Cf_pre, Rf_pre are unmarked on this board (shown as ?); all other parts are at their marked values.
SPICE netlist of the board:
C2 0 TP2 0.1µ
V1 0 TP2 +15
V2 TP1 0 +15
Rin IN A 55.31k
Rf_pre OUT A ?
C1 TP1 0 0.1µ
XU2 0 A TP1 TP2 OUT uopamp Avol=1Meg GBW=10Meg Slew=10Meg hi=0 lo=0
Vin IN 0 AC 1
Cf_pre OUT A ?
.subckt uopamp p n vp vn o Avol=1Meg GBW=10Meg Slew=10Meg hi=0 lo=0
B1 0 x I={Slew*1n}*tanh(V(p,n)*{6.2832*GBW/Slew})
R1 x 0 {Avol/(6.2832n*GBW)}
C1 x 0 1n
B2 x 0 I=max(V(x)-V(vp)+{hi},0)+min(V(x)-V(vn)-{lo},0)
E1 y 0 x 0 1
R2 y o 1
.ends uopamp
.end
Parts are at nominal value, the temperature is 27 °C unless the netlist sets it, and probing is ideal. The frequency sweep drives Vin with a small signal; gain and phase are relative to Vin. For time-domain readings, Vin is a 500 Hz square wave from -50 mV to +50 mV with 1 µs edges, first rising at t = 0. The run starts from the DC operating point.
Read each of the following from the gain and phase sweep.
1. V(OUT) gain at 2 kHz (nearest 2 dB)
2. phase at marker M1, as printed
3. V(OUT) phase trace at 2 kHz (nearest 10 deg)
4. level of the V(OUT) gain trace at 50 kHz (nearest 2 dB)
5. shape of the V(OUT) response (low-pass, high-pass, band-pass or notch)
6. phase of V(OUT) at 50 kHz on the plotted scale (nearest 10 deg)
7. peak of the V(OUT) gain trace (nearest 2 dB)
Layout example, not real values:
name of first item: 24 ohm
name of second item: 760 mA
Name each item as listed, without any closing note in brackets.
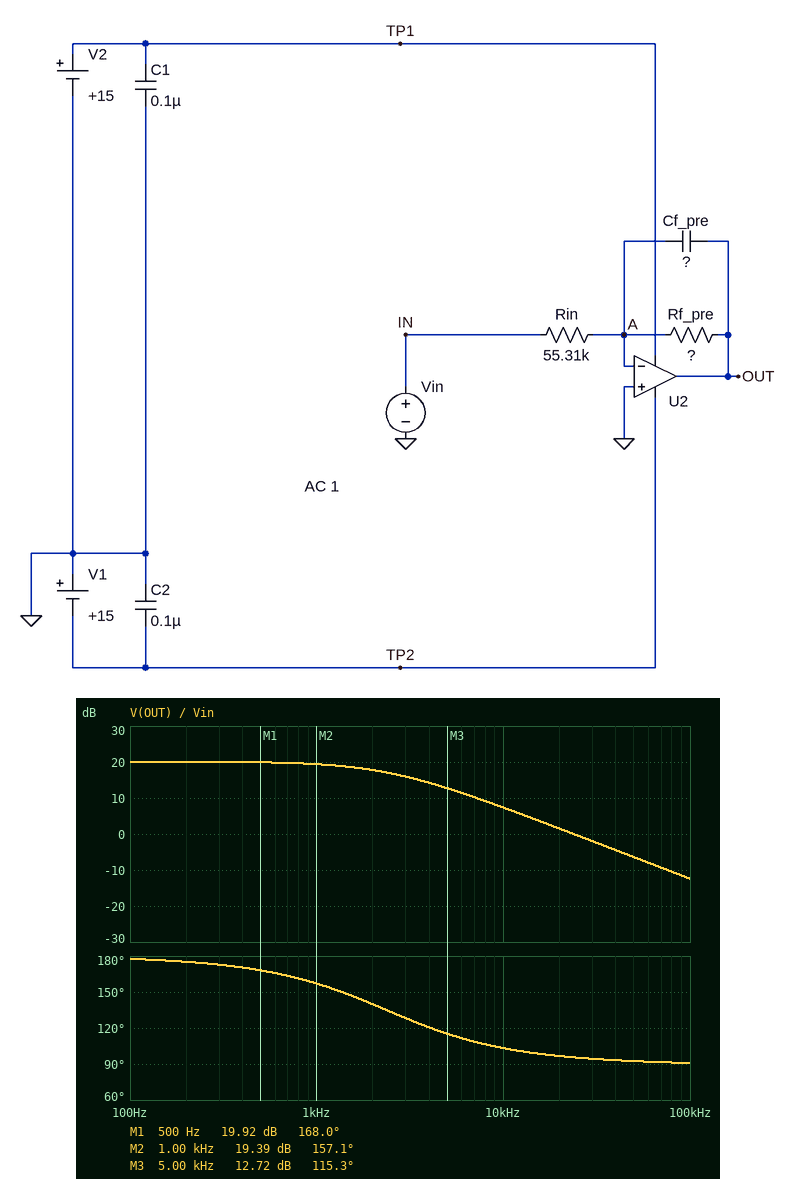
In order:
V(OUT) gain at 2 kHz: 18 dB
phase at marker M1, as printed: 168.0 deg
V(OUT) phase trace at 2 kHz: 140 deg
level of the V(OUT) gain trace at 50 kHz: -6 dB
shape of the V(OUT) response: low-pass
phase of V(OUT) at 50 kHz on the plotted scale: 90 deg
peak of the V(OUT) gain trace: 20 dB
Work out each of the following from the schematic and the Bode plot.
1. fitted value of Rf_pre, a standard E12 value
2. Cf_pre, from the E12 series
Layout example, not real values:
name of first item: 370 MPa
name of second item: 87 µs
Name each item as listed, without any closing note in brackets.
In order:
fitted value of Rf_pre, a standard E12 value: 560 kΩ
Cf_pre, from the E12 series: 120 pF
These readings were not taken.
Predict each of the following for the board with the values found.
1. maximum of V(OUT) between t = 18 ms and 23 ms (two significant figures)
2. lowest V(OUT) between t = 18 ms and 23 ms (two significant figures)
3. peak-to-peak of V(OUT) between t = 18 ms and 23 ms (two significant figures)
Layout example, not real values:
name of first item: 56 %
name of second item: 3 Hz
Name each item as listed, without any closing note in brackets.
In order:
maximum of V(OUT) between t = 18 ms and 23 ms: 510 mV
lowest V(OUT) between t = 18 ms and 23 ms: -510 mV
peak-to-peak of V(OUT) between t = 18 ms and 23 ms: 1.0 V
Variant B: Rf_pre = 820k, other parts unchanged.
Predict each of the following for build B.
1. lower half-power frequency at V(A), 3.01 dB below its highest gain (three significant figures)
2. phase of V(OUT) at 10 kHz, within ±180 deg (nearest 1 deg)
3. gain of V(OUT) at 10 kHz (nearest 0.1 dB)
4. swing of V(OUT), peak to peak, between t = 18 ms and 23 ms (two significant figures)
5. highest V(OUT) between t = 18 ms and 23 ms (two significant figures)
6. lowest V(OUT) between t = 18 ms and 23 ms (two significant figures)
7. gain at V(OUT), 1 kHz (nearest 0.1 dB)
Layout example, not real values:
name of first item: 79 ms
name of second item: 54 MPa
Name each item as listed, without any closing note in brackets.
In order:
lower half-power frequency at V(A), 3.01 dB below its highest gain: 1.61 kHz
phase of V(OUT) at 10 kHz, within ±180 deg: 99 deg
gain of V(OUT) at 10 kHz: 7.5 dB
swing of V(OUT), peak to peak, between t = 18 ms and 23 ms: 1.5 V
highest V(OUT) between t = 18 ms and 23 ms: 740 mV
lowest V(OUT) between t = 18 ms and 23 ms: -740 mV
gain at V(OUT), 1 kHz: 22.0 dB
